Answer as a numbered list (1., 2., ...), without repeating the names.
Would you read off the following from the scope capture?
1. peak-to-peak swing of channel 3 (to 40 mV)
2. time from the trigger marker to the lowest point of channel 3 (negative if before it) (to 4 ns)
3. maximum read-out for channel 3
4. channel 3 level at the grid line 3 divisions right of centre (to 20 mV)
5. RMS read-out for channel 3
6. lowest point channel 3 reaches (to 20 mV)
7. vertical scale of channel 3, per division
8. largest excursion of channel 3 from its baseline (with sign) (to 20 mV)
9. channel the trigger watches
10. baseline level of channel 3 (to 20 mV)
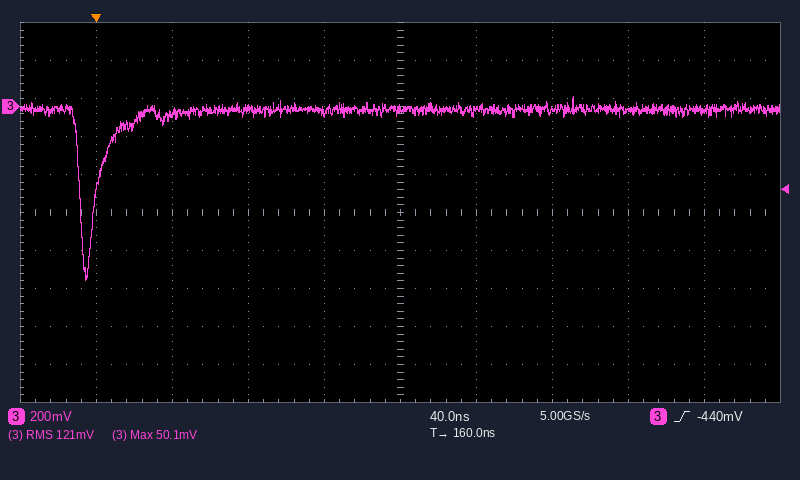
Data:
1. 960 mV
2. -4 ns
3. 50.1 mV
4. -20 mV
5. 121 mV
6. -920 mV
7. 200 mV
8. -900 mV
9. channel 3
10. -20 mV
